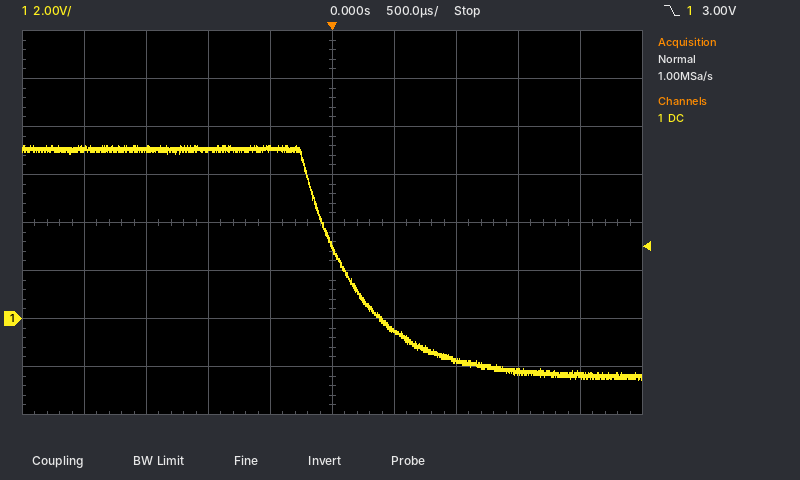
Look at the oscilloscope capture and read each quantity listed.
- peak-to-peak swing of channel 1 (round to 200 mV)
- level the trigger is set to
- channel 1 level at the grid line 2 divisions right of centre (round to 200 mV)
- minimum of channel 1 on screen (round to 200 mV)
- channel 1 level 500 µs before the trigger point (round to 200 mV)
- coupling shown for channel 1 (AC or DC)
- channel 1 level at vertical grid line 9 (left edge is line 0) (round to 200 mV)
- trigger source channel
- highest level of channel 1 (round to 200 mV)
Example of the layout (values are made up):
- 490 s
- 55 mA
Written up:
- 9.8 V
- 3.00 V
- -1.8 V
- -2.6 V
- 7.0 V
- DC
- -2.4 V
- channel 1
- 7.2 V
